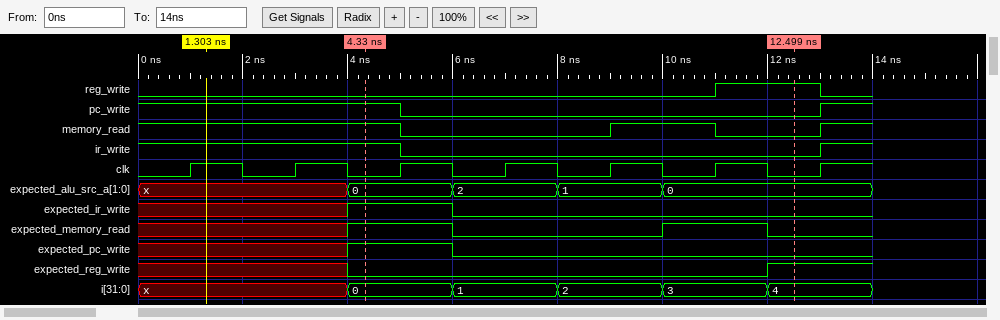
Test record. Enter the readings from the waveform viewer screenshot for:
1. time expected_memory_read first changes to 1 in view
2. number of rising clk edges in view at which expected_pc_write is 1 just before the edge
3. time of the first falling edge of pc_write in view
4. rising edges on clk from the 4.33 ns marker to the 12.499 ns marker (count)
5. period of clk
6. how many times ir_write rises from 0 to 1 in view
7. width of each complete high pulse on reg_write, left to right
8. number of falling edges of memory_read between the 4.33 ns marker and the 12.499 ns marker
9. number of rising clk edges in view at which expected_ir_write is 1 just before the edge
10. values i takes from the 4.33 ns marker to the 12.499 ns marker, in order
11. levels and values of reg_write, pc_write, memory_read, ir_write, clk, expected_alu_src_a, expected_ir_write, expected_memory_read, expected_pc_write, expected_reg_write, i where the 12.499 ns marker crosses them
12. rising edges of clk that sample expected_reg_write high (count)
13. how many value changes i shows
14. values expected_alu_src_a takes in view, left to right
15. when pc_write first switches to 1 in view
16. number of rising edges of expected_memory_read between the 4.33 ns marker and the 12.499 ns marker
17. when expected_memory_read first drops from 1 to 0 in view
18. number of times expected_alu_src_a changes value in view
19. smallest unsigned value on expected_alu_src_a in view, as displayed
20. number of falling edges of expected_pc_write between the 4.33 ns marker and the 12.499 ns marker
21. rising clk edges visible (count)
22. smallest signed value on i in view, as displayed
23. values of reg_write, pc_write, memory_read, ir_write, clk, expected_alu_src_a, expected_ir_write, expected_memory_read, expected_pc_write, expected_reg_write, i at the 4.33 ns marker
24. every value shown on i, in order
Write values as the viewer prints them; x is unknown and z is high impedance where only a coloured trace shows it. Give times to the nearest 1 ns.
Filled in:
4 ns
1
5 ns
4
2 ns
1
2 ns
2
1
0, 1, 2, 3, 4
reg_write=1, pc_write=0, memory_read=0, ir_write=0, clk=0, expected_alu_src_a=0, expected_ir_write=0, expected_memory_read=0, expected_pc_write=0, expected_reg_write=1, i=4
1
5
x, 0, 2, 1, 0
13 ns
1
6 ns
4
0
1
7
0
reg_write=0, pc_write=1, memory_read=1, ir_write=1, clk=0, expected_alu_src_a=0, expected_ir_write=1, expected_memory_read=1, expected_pc_write=1, expected_reg_write=0, i=0
x, 0, 1, 2, 3, 4
